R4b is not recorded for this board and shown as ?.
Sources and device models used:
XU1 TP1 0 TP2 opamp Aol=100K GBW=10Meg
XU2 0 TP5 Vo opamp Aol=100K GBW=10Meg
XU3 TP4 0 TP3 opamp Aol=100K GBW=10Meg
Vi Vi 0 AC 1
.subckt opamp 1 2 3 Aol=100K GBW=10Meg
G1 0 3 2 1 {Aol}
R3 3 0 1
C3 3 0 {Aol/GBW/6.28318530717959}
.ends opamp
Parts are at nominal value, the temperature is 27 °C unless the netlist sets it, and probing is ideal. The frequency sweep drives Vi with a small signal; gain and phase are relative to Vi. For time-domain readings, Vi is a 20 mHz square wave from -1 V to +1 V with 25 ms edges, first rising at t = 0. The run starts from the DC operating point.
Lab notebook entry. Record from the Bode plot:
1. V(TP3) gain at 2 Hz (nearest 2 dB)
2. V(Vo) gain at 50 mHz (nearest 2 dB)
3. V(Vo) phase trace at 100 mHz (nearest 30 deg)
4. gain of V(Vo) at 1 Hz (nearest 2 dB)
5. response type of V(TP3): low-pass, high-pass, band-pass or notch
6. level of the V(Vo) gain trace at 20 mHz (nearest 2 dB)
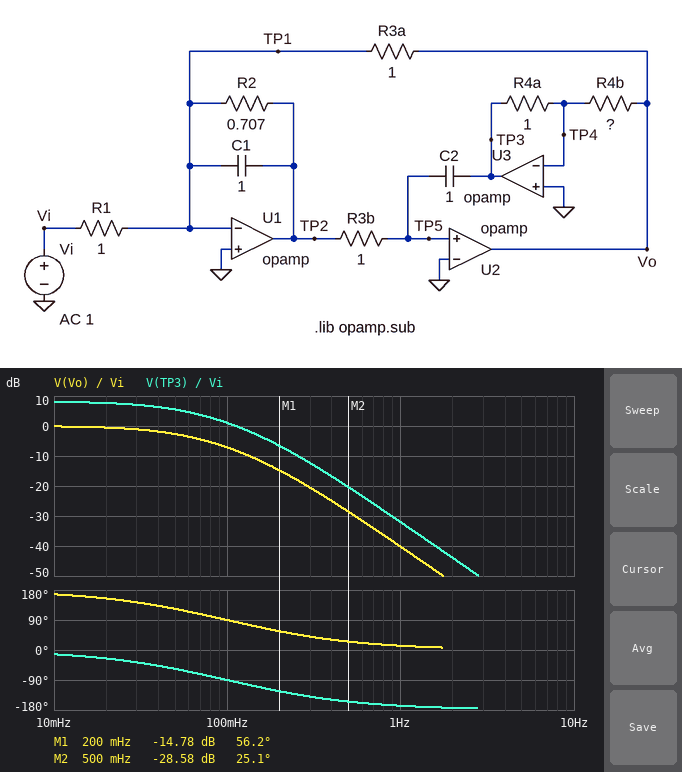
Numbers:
-44 dB
-2 dB
90 deg
-40 dB
low-pass
0 dB
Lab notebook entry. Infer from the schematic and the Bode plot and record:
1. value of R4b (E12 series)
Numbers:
0.39 Ω
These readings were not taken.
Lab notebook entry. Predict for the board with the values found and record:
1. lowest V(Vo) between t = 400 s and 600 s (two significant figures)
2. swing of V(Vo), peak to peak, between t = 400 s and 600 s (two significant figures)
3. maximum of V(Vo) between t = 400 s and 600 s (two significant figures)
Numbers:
-1.0 V
2.0 V
1.0 V
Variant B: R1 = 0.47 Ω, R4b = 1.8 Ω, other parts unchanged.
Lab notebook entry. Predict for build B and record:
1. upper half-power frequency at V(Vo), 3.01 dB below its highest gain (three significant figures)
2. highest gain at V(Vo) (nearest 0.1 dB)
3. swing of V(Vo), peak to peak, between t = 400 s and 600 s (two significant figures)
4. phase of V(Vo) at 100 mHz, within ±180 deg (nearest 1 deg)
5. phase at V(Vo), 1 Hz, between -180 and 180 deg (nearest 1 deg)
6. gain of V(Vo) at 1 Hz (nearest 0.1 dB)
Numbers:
247 mHz
7.5 dB
5.5 V
148 deg
13 deg
-20.1 dB
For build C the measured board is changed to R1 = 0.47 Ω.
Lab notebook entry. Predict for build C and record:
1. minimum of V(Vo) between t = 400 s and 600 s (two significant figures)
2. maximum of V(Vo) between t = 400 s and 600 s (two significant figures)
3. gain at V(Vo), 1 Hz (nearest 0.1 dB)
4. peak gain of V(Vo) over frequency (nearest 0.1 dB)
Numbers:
-2.1 V
2.1 V
-33.7 dB
6.6 dB
